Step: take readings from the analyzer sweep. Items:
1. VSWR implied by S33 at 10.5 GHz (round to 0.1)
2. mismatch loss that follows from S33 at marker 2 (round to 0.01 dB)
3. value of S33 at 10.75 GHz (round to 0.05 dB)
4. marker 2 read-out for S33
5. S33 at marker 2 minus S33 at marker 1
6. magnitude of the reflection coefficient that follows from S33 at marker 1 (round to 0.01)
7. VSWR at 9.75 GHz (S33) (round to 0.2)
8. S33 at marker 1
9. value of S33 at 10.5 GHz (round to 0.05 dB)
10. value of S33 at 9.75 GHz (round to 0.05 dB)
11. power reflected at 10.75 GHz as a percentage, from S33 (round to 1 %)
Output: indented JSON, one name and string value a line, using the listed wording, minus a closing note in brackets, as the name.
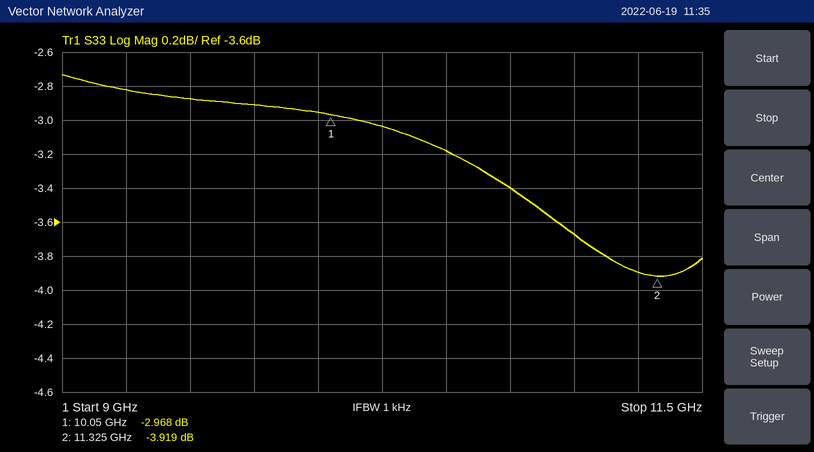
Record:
{
  "VSWR implied by S33 at 10.5 GHz": "5.5",
  "mismatch loss that follows from S33 at marker 2": "2.26 dB",
  "value of S33 at 10.75 GHz": "-3.40 dB",
  "marker 2 read-out for S33": "-3.919 dB",
  "S33 at marker 2 minus S33 at marker 1": "-0.951 dB",
  "magnitude of the reflection coefficient that follows from S33 at marker 1": "0.71",
  "VSWR at 9.75 GHz (S33)": "6.0",
  "S33 at marker 1": "-2.968 dB",
  "value of S33 at 10.5 GHz": "-3.20 dB",
  "value of S33 at 9.75 GHz": "-2.90 dB",
  "power reflected at 10.75 GHz as a percentage, from S33": "46 %"
}
